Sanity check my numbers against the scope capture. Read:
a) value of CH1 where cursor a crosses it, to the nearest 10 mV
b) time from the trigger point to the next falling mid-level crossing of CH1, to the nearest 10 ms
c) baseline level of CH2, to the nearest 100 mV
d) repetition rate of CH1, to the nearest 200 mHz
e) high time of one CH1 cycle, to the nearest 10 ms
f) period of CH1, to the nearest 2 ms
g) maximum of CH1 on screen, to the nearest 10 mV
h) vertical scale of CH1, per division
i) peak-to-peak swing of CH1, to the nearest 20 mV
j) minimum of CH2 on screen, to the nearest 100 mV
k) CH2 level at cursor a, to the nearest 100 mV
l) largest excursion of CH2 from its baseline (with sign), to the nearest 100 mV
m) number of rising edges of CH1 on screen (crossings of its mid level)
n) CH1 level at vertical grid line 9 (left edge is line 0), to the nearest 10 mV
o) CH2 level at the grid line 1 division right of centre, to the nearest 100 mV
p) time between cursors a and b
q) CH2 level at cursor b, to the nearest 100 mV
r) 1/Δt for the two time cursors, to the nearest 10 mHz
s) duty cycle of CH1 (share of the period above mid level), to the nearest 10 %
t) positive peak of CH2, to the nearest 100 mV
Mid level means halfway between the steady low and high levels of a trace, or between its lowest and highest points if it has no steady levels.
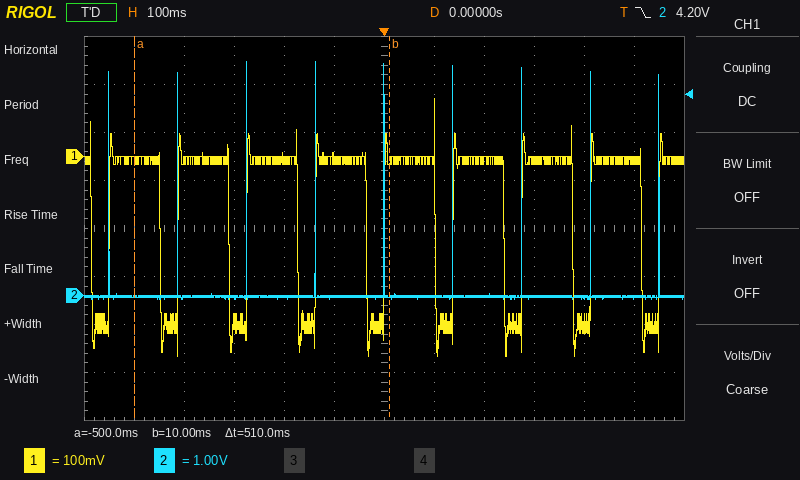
-10 mV
100 ms
0.0 V
7.2 Hz
100 ms
138 ms
120 mV
100 mV
540 mV
-100 mV
0.0 V
+4.9 V
9
-10 mV
0.0 V
510 ms
0.0 V
1.96 Hz
70 %
4.9 V
